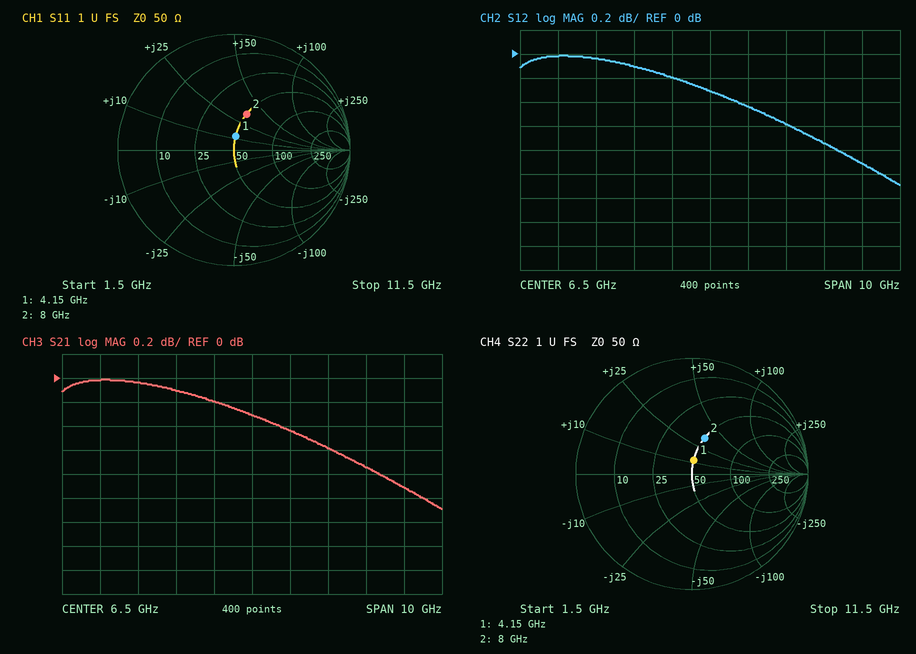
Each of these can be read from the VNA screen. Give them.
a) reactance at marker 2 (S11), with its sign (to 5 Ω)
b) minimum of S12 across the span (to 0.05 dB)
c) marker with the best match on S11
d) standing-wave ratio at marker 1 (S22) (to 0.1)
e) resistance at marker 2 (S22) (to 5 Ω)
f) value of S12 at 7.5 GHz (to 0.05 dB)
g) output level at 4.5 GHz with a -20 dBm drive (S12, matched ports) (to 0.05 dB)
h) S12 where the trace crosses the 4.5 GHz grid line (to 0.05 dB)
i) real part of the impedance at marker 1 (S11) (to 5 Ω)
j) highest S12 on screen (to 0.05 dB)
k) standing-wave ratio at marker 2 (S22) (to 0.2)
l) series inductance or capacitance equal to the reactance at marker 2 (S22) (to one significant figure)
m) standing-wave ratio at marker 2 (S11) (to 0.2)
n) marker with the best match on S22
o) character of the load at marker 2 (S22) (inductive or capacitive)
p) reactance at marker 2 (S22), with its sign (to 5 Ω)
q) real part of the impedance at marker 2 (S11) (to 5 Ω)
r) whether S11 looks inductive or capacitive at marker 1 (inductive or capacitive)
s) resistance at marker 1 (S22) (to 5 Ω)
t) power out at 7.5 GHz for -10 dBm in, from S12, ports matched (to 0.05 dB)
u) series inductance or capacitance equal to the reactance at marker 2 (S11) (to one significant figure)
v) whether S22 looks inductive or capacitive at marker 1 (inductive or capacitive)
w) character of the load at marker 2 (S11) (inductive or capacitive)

+35 Ω
-1.10 dB
marker 1
1.3
50 Ω
-0.45 dB
-20.10 dBm
-0.10 dB
50 Ω
0.00 dB
2.0
700 pH
2.0
marker 1
inductive
+35 Ω
50 Ω
inductive
50 Ω
-10.45 dBm
700 pH
inductive
inductive
